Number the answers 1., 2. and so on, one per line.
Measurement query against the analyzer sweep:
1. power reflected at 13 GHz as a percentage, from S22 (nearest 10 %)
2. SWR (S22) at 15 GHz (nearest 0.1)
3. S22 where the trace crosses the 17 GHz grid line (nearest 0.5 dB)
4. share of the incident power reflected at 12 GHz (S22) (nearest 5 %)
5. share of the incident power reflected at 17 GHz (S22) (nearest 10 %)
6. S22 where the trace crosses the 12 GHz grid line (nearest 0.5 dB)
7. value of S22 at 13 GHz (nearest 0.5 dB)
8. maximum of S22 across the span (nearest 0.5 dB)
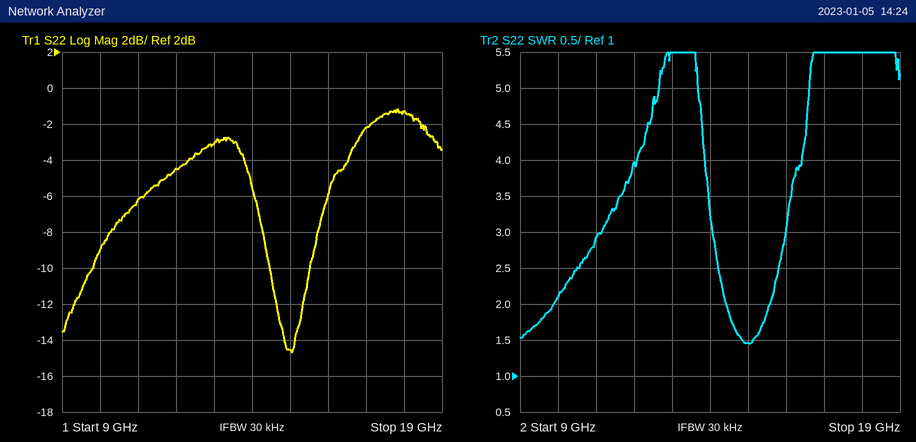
1. 50 %
2. 1.5
3. -2.0 dB
4. 35 %
5. 60 %
6. -4.5 dB
7. -3.0 dB
8. -1.0 dB
